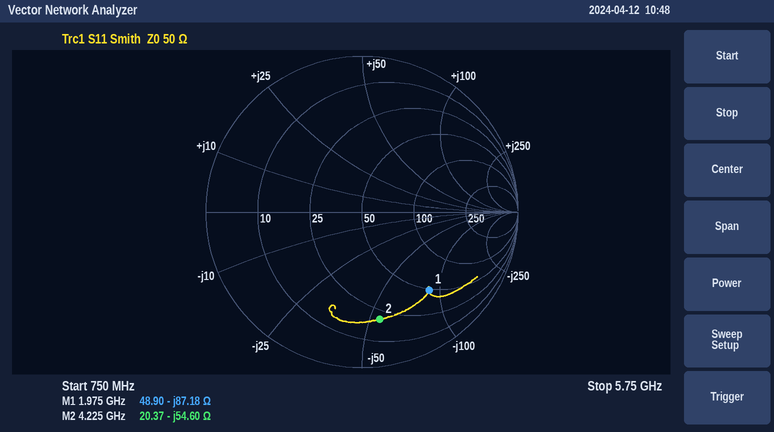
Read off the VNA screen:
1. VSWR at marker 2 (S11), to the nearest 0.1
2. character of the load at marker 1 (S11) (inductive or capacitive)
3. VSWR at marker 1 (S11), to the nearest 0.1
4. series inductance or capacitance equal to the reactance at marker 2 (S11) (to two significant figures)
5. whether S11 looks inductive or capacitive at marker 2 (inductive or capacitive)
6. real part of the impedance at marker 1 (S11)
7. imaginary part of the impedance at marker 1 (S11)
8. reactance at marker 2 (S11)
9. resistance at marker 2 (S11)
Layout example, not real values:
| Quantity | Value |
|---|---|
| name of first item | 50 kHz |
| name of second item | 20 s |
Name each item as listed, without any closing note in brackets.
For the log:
| Quantity | Value |
|---|---|
| VSWR at marker 2 (S11), to the nearest 0.1 | 5.6 |
| character of the load at marker 1 (S11) | capacitive |
| VSWR at marker 1 (S11), to the nearest 0.1 | 4.9 |
| series inductance or capacitance equal to the reactance at marker 2 (S11) | 690 fF |
| whether S11 looks inductive or capacitive at marker 2 | capacitive |
| real part of the impedance at marker 1 | 48.90 Ω |
| imaginary part of the impedance at marker 1 | -87.18 Ω |
| reactance at marker 2 | -54.60 Ω |
| resistance at marker 2 | 20.37 Ω |
